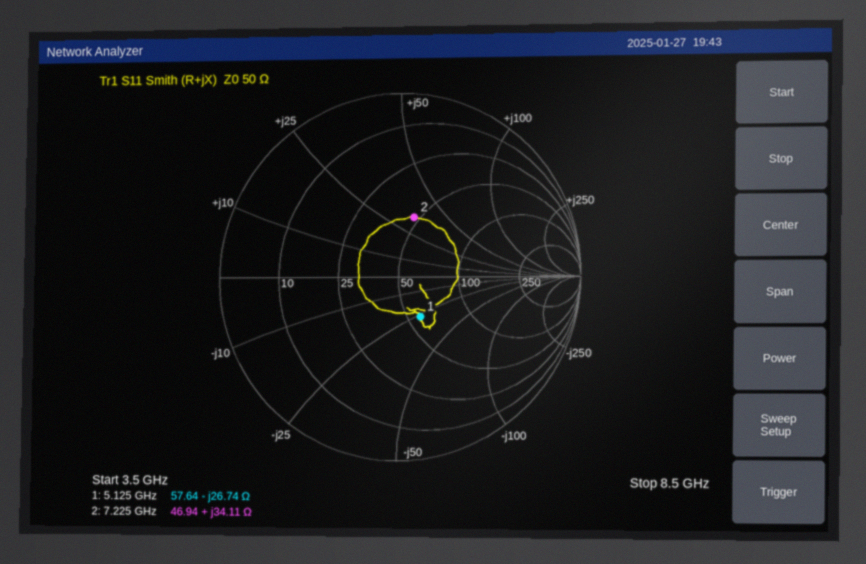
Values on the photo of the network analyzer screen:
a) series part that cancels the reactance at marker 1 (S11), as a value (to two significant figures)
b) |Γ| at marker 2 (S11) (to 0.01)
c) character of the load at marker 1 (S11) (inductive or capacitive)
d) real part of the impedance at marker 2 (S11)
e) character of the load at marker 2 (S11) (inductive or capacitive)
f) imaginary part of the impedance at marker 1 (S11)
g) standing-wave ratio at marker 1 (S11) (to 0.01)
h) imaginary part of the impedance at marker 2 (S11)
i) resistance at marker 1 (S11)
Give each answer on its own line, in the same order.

830 pH
0.33
capacitive
46.94 Ω
inductive
-26.74 Ω
1.67
+34.11 Ω
57.64 Ω
